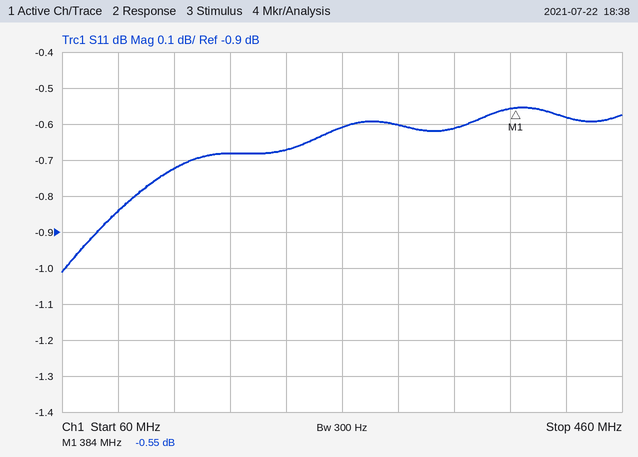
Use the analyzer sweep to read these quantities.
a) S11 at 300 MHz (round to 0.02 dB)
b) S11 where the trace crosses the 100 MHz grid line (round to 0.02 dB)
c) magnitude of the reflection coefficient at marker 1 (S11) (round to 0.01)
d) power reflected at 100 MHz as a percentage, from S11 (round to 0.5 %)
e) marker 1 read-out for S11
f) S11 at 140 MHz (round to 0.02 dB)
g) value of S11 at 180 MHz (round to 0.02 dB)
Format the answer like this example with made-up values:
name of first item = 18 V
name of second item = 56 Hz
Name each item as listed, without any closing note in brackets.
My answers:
S11 at 300 MHz = -0.60 dB
S11 where the trace crosses the 100 MHz grid line = -0.84 dB
magnitude of the reflection coefficient at marker 1 (S11) = 0.94
power reflected at 100 MHz as a percentage, from S11 = 82.5 %
marker 1 read-out for S11 = -0.55 dB
S11 at 140 MHz = -0.72 dB
value of S11 at 180 MHz = -0.68 dB
